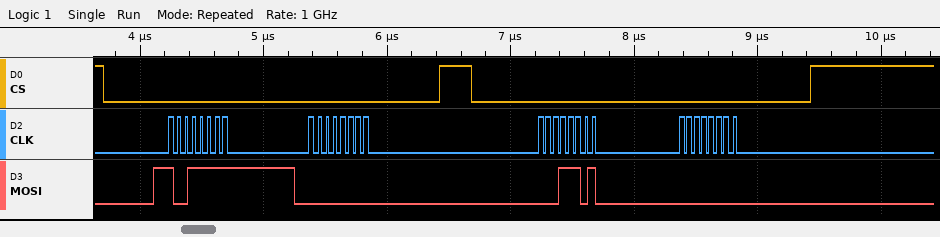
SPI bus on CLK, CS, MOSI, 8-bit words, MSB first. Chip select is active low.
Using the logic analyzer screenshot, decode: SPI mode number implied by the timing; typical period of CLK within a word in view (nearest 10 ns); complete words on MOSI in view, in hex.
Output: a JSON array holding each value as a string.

["0", "60 ns", "9F, 00, 1D, 00"]
